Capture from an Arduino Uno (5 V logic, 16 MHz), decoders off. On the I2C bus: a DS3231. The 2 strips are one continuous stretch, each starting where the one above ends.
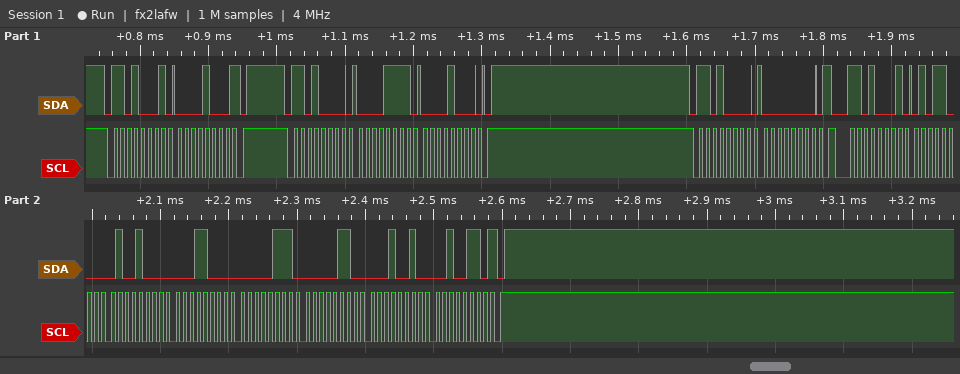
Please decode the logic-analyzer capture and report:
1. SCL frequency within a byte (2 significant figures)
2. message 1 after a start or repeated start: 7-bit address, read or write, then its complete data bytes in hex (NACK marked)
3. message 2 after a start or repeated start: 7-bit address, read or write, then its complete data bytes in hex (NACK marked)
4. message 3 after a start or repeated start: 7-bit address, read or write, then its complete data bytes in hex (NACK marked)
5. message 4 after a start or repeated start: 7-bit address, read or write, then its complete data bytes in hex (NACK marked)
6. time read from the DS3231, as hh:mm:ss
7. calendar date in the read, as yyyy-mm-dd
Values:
100 kHz
0x68 read: 08 NACK
0x68 write: 0F 08
0x68 write: 00
0x68 read: 58 48 18 07 06 12 26 NACK
18:48:58
2026-12-06
